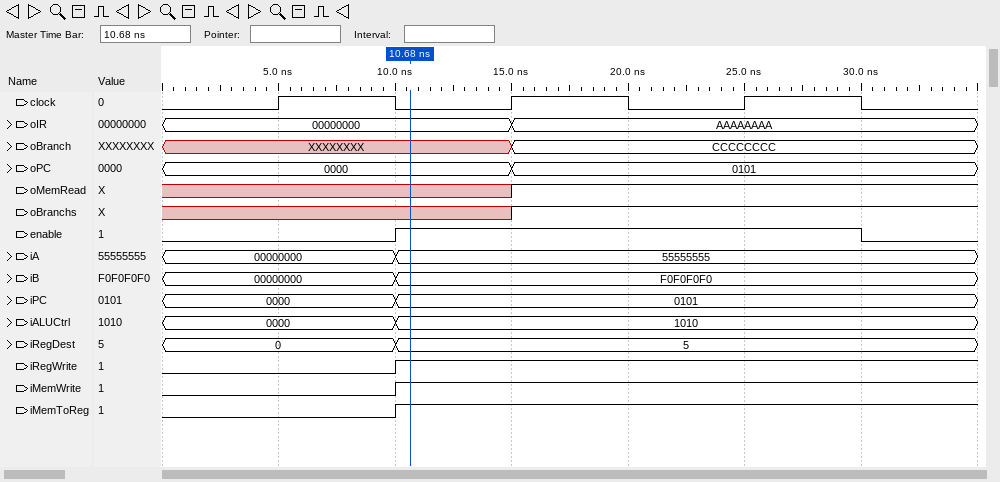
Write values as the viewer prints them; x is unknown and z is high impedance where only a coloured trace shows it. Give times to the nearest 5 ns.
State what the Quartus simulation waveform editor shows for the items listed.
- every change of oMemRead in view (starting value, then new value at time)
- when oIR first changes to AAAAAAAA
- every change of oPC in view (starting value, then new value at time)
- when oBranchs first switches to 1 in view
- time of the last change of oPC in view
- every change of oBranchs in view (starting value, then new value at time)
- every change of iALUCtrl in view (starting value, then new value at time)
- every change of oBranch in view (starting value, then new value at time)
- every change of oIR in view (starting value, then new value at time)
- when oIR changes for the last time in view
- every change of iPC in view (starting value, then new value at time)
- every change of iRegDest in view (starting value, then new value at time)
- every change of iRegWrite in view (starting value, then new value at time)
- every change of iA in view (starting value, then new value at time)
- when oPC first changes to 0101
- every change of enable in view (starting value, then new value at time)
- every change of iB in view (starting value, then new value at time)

x, 1 at 15 ns
15 ns
0000, 0101 at 15 ns
15 ns
15 ns
x, 1 at 15 ns
0000, 1010 at 10 ns
XXXXXXXX, CCCCCCCC at 15 ns
00000000, AAAAAAAA at 15 ns
15 ns
0000, 0101 at 10 ns
0, 5 at 10 ns
0, 1 at 10 ns
00000000, 55555555 at 10 ns
15 ns
0, 1 at 10 ns, 0 at 30 ns
00000000, F0F0F0F0 at 10 ns
